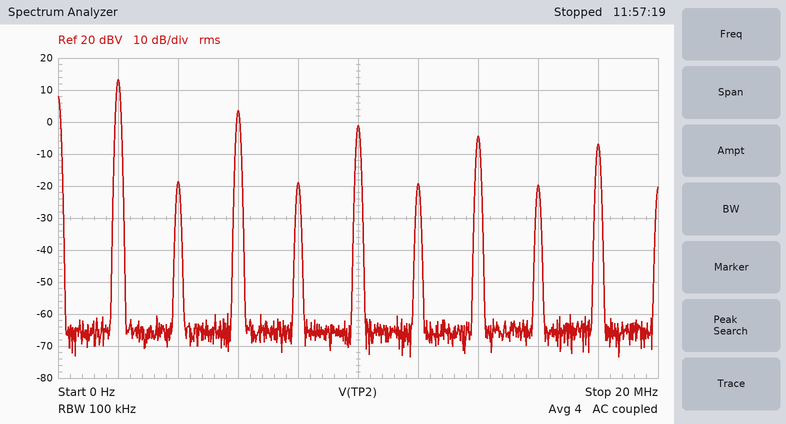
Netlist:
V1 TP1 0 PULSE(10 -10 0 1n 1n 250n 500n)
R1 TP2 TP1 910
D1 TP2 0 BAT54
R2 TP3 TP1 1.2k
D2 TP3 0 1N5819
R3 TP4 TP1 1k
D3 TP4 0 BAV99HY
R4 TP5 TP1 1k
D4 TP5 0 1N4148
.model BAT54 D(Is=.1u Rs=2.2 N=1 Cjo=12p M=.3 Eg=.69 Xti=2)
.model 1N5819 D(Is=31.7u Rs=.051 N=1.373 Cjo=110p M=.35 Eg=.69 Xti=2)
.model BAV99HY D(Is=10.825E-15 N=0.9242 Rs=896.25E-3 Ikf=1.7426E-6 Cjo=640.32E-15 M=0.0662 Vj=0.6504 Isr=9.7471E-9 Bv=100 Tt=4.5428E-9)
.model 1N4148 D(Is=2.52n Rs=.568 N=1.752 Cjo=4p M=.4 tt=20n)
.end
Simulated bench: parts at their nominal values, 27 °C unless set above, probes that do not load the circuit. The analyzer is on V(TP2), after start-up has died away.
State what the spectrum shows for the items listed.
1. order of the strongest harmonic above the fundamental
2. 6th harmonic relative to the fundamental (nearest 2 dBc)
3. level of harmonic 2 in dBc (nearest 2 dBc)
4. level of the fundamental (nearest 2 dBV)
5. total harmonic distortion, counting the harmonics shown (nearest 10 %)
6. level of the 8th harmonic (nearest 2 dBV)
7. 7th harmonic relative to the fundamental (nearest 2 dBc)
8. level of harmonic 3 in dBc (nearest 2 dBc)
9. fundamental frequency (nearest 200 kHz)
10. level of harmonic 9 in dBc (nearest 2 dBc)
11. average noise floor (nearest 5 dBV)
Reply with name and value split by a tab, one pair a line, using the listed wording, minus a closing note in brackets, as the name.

order of the strongest harmonic above the fundamental	3
6th harmonic relative to the fundamental	-32 dBc
level of harmonic 2 in dBc	-32 dBc
level of the fundamental	14 dBV
total harmonic distortion, counting the harmonics shown	40 %
level of the 8th harmonic	-20 dBV
7th harmonic relative to the fundamental	-18 dBc
level of harmonic 3 in dBc	-10 dBc
fundamental frequency	2.0 MHz
level of harmonic 9 in dBc	-20 dBc
average noise floor	-65 dBV
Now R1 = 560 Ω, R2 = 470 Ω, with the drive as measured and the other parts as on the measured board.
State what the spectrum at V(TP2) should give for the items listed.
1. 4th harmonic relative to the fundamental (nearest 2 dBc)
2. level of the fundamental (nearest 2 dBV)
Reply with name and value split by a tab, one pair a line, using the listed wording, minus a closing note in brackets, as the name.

4th harmonic relative to the fundamental	-38 dBc
level of the fundamental	14 dBV
